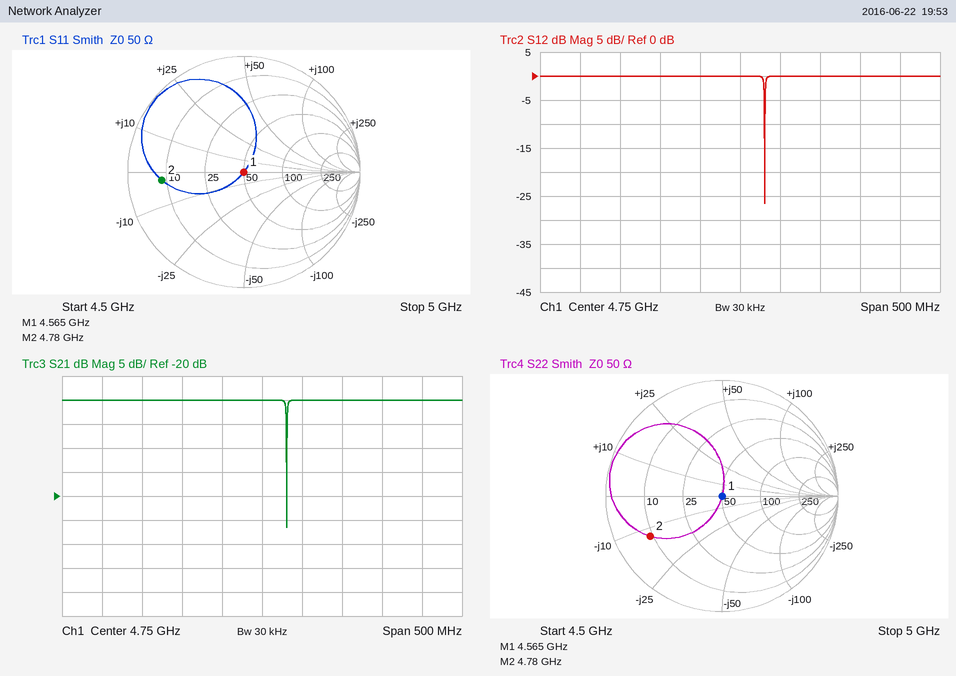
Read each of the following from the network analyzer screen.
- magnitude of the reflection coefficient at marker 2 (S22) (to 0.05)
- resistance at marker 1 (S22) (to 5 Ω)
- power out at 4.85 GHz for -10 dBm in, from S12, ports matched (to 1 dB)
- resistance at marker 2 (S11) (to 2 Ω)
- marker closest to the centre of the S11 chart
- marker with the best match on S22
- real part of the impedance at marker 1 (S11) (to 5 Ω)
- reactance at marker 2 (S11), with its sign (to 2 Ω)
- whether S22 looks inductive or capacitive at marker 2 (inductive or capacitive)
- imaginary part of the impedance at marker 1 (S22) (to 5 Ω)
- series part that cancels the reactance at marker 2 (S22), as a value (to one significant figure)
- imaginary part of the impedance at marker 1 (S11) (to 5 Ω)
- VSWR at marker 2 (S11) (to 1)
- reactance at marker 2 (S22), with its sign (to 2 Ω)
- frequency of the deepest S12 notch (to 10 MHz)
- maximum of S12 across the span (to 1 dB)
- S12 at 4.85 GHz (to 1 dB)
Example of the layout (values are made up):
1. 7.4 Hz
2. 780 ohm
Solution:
1. 0.70
2. 50 Ω
3. -10 dBm
4. 8 Ω
5. marker 1
6. marker 1
7. 50 Ω
8. -2 Ω
9. capacitive
10. 0 Ω
11. 400 pH
12. 0 Ω
13. 6
14. -12 Ω
15. 4.78 GHz
16. 0 dB
17. 0 dB
